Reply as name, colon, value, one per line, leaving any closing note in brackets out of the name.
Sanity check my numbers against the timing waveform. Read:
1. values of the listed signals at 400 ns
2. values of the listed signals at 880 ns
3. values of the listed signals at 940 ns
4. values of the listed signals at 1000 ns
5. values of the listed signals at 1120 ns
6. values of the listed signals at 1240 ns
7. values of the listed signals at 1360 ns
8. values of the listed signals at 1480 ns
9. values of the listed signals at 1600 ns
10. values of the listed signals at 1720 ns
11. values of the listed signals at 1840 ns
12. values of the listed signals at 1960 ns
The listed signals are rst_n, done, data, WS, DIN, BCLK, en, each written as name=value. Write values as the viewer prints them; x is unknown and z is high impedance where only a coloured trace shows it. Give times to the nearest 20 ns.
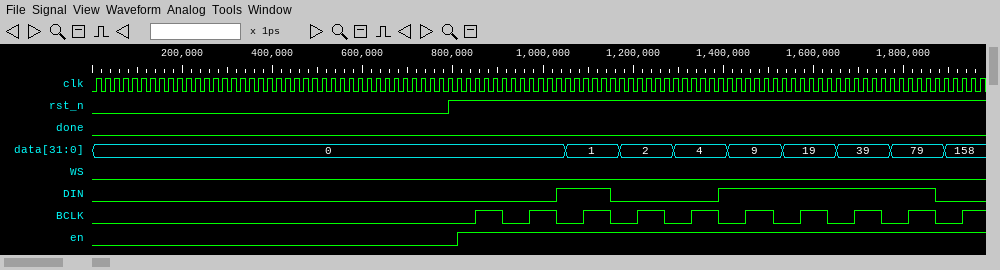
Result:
values of the listed signals at 400 ns: rst_n=0, done=0, data=0, WS=0, DIN=0, BCLK=0, en=0
values of the listed signals at 880 ns: rst_n=1, done=0, data=0, WS=0, DIN=0, BCLK=1, en=1
values of the listed signals at 940 ns: rst_n=1, done=0, data=0, WS=0, DIN=0, BCLK=0, en=1
values of the listed signals at 1000 ns: rst_n=1, done=0, data=0, WS=0, DIN=0, BCLK=1, en=1
values of the listed signals at 1120 ns: rst_n=1, done=0, data=1, WS=0, DIN=1, BCLK=1, en=1
values of the listed signals at 1240 ns: rst_n=1, done=0, data=2, WS=0, DIN=0, BCLK=1, en=1
values of the listed signals at 1360 ns: rst_n=1, done=0, data=4, WS=0, DIN=0, BCLK=1, en=1
values of the listed signals at 1480 ns: rst_n=1, done=0, data=9, WS=0, DIN=1, BCLK=1, en=1
values of the listed signals at 1600 ns: rst_n=1, done=0, data=19, WS=0, DIN=1, BCLK=1, en=1
values of the listed signals at 1720 ns: rst_n=1, done=0, data=39, WS=0, DIN=1, BCLK=1, en=1
values of the listed signals at 1840 ns: rst_n=1, done=0, data=79, WS=0, DIN=1, BCLK=1, en=1
values of the listed signals at 1960 ns: rst_n=1, done=0, data=158, WS=0, DIN=0, BCLK=1, en=1
